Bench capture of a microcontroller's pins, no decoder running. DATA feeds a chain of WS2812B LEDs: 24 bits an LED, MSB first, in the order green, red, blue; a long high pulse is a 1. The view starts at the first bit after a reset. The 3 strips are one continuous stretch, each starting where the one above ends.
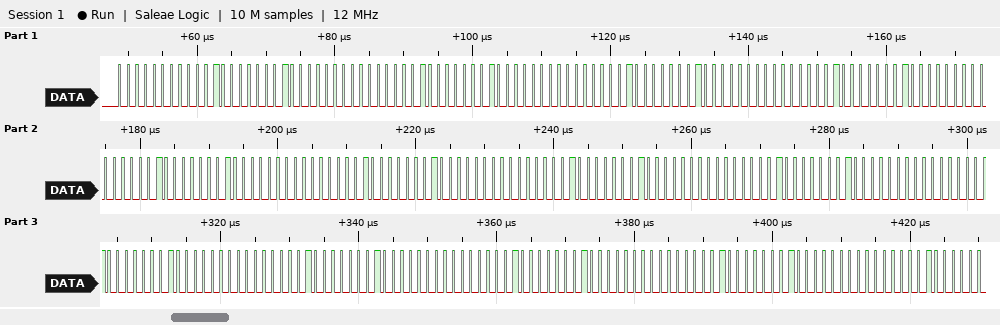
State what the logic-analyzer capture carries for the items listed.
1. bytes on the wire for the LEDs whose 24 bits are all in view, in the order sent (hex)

00 10 10 00 10 10 00 10 10 00 10 10 00 10 10 00 10 10 00 10 10 00 10 10 00 10 10 00 10 10 00 10 10 00 10 10
